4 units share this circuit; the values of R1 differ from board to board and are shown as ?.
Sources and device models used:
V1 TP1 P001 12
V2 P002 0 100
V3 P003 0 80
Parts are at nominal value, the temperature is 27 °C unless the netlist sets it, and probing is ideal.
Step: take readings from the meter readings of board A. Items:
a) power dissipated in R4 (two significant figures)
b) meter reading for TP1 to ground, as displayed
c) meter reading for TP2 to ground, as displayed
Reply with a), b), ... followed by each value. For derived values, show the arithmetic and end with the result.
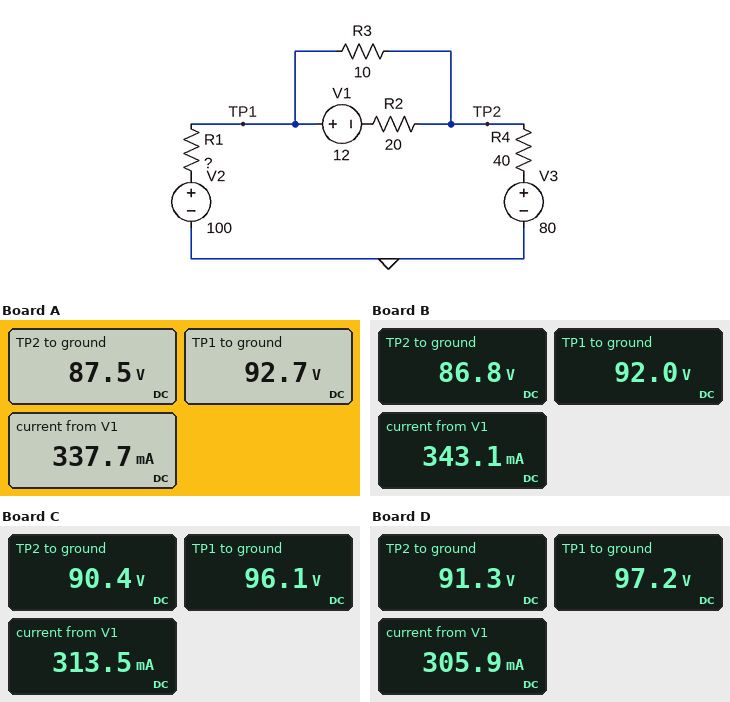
a) (87.5 V - 80 V)^2 / 40 Ω = 1.4 W
b) 92.7 V
c) 87.5 V
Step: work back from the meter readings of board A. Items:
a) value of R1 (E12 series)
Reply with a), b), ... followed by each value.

a) 39 Ω
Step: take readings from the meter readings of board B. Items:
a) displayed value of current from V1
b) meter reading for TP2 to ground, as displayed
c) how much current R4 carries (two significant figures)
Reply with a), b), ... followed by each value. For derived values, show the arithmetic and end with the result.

a) 343.1 mA
b) 86.8 V
c) (86.8 V - 80 V) / 40 Ω = 170 mA
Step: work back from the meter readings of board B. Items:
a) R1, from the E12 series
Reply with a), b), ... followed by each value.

a) 47 Ω
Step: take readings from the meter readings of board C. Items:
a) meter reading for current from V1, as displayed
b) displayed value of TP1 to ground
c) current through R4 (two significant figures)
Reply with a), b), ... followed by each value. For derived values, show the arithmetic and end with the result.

a) 313.5 mA
b) 96.1 V
c) (90.4 V - 80 V) / 40 Ω = 260 mA
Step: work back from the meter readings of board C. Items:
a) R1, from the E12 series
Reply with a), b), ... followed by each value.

a) 15 Ω
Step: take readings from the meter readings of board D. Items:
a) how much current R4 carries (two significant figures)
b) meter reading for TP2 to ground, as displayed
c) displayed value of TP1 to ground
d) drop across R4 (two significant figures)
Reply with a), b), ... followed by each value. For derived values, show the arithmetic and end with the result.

a) (91.3 V - 80 V) / 40 Ω = 280 mA
b) 91.3 V
c) 97.2 V
d) 91.3 V - 80 V = 11 V
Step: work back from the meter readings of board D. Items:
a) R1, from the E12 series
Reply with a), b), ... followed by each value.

a) 10 Ω
